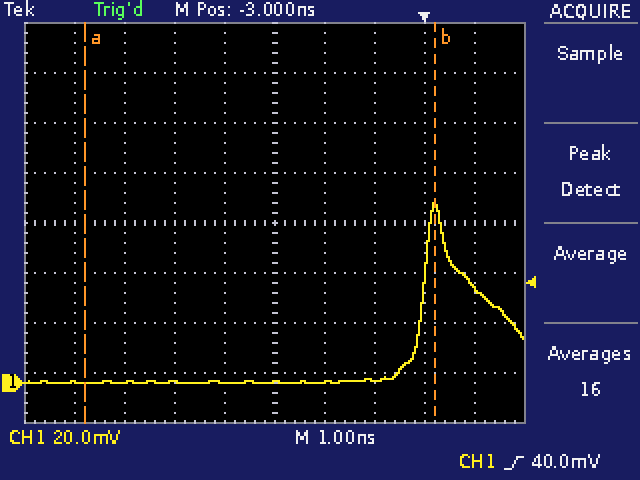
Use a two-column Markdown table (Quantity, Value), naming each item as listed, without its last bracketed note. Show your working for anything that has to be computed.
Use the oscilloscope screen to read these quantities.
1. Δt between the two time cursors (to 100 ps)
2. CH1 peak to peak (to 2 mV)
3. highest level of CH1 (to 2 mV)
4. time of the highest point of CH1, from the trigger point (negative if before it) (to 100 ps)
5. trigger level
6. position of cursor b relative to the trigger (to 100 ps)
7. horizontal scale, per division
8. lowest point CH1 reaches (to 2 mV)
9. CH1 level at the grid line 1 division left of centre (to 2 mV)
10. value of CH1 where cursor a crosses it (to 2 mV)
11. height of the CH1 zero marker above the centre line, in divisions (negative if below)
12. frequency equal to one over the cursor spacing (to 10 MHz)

| Quantity | Value |
|---|---|
| Δt between the two time cursors | 7.0 ns |
| CH1 peak to peak | 72 mV − (0 mV) = 72 mV |
| highest level of CH1 | 72 mV |
| time of the highest point of CH1, from the trigger point (negative if before it) | +200 ps |
| trigger level | 40.0 mV |
| position of cursor b relative to the trigger | +200 ps |
| horizontal scale, per division | 1 ns |
| lowest point CH1 reaches | 0 mV |
| CH1 level at the grid line 1 division left of centre | 0 mV |
| value of CH1 where cursor a crosses it | 0 mV |
| height of the CH1 zero marker above the centre line, in divisions | -3.2 div |
| frequency equal to one over the cursor spacing | 1 / 7.0 ns ≈ 140 MHz |
